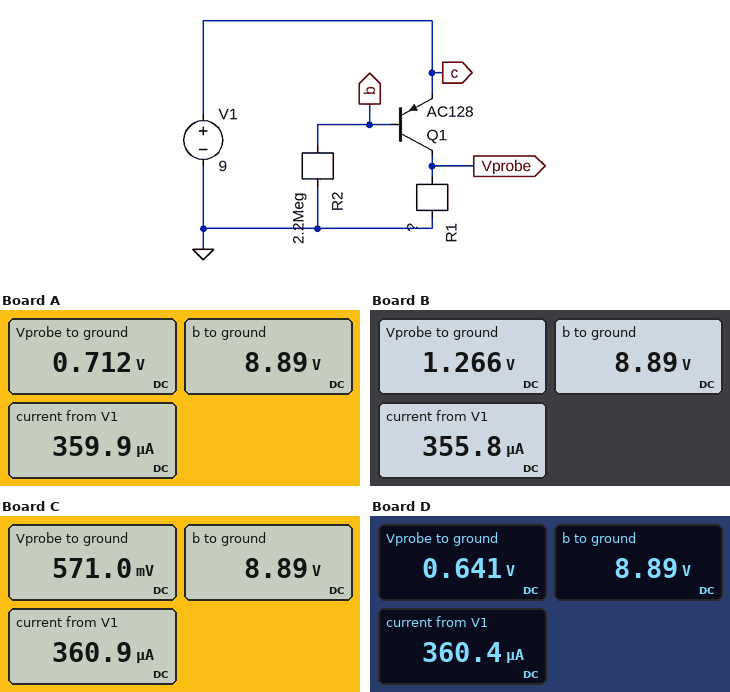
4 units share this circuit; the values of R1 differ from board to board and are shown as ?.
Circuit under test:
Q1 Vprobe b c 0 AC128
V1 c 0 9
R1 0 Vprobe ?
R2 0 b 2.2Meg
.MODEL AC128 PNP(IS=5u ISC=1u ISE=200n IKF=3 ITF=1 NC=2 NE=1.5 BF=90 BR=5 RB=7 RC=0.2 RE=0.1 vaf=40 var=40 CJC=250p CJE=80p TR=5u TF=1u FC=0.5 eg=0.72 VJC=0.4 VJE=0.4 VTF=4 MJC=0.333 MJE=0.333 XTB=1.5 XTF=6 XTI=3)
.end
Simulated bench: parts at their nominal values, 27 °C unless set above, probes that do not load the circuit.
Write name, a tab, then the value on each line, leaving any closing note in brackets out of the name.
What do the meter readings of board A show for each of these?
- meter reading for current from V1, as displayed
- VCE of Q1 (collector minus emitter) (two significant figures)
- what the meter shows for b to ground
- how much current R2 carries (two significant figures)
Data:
meter reading for current from V1, as displayed	359.9 µA
VCE of Q1 (collector minus emitter)	-8.3 V
what the meter shows for b to ground	8.89 V
how much current R2 carries	4.0 µA
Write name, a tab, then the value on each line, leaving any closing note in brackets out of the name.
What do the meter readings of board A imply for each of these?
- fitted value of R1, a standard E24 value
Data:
fitted value of R1, a standard E24 value	2 kΩ
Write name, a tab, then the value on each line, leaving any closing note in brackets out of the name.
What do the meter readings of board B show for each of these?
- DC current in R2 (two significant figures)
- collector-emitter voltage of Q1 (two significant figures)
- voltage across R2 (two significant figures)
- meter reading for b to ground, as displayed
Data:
DC current in R2	4.0 µA
collector-emitter voltage of Q1	-7.7 V
voltage across R2	8.9 V
meter reading for b to ground, as displayed	8.89 V
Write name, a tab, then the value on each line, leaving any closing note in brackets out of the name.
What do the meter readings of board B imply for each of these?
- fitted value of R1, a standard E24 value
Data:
fitted value of R1, a standard E24 value	3.6 kΩ
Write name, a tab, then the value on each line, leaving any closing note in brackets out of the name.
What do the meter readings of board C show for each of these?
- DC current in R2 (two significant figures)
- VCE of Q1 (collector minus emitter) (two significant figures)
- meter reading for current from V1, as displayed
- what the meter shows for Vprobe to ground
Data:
DC current in R2	4.0 µA
VCE of Q1 (collector minus emitter)	-8.4 V
meter reading for current from V1, as displayed	360.9 µA
what the meter shows for Vprobe to ground	571.0 mV
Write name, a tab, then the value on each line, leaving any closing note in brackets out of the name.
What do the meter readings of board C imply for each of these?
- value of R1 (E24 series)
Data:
value of R1	1.6 kΩ
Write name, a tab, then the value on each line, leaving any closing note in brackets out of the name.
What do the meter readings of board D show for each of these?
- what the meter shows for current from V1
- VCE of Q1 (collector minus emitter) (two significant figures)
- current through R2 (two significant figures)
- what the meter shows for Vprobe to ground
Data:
what the meter shows for current from V1	360.4 µA
VCE of Q1 (collector minus emitter)	-8.4 V
current through R2	4.0 µA
what the meter shows for Vprobe to ground	0.641 V
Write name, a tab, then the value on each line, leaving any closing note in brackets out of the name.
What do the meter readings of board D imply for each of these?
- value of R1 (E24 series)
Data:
value of R1	1.8 kΩ
